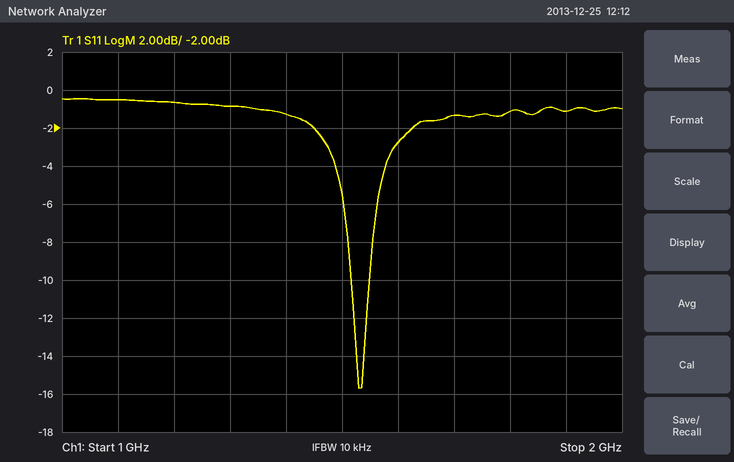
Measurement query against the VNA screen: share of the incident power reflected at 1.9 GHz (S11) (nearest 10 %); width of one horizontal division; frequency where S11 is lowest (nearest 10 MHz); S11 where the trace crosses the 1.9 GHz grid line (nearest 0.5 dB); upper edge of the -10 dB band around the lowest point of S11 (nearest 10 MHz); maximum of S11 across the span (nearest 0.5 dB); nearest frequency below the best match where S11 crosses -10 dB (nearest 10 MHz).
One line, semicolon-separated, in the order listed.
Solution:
80 %; 100 MHz; 1.53 GHz; -1.0 dB; 1.55 GHz; -0.5 dB; 1.52 GHz
